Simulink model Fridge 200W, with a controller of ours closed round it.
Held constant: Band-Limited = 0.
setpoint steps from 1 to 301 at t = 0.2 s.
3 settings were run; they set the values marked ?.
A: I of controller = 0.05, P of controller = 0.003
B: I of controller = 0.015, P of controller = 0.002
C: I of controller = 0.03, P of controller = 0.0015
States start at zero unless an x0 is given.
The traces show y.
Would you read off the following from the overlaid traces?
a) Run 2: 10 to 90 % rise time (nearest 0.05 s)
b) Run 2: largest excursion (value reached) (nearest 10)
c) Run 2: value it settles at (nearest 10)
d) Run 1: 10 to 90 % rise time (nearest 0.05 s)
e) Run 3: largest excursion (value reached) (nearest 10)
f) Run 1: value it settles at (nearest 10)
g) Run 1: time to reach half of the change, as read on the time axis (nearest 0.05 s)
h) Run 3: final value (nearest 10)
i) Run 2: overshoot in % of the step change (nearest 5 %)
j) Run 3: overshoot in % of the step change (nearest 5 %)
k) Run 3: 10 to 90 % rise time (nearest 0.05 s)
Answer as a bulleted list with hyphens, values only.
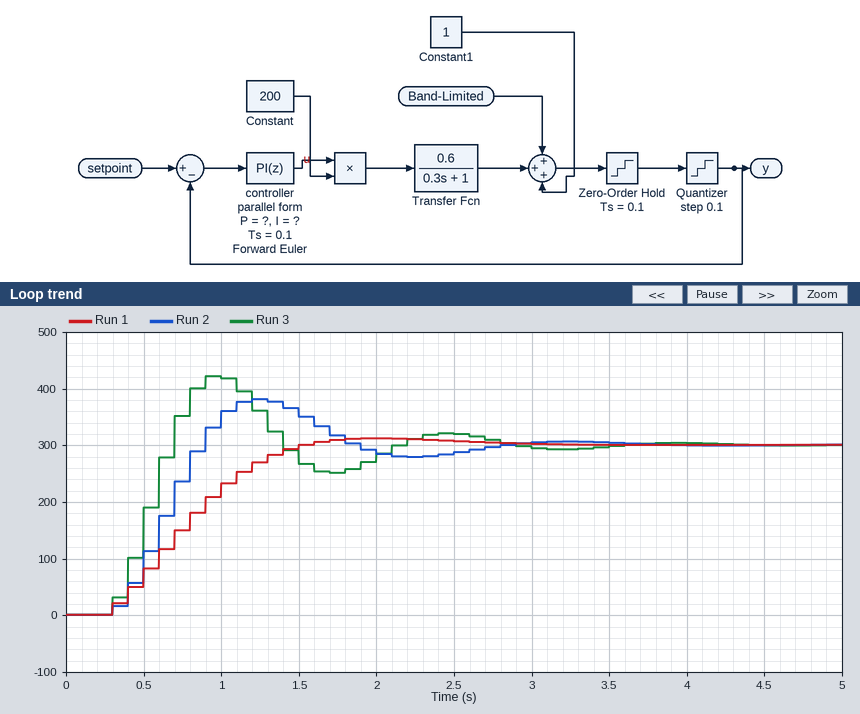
- 0.40 s
- 380
- 300
- 0.90 s
- 420
- 300
- 0.80 s
- 300
- 25 %
- 40 %
- 0.30 s
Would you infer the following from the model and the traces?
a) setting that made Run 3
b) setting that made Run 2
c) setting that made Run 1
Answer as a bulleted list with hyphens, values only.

- A
- C
- B
